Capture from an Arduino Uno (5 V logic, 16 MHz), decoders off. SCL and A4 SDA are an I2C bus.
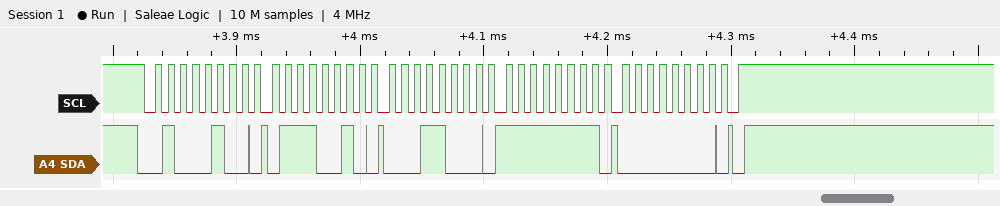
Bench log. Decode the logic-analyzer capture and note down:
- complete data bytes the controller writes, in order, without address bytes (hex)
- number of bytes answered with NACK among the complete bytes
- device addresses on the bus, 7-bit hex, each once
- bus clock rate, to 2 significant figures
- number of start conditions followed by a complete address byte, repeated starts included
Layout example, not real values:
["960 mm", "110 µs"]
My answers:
["72 18 FF 00", "0", "0x22", "100 kHz", "1"]
